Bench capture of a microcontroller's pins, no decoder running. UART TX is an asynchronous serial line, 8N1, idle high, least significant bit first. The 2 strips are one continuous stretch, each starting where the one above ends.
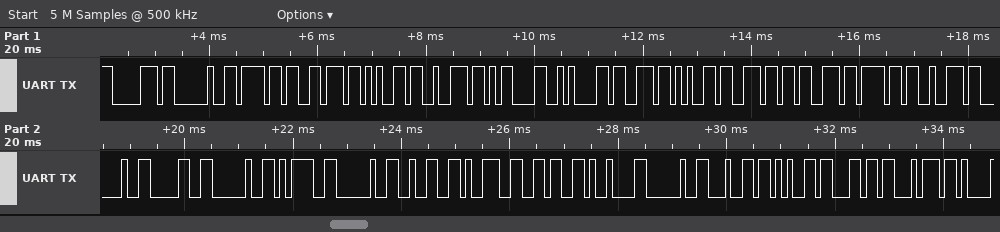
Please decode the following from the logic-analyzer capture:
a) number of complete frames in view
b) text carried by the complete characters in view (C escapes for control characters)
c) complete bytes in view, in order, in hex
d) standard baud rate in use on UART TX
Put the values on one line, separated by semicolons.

28; "p over\r\nsensor 0 = 296\t delt"; 70 20 6F 76 65 72 0D 0A 73 65 6E 73 6F 72 20 30 20 3D 20 32 39 36 09 20 64 65 6C 74; 9600 baud
